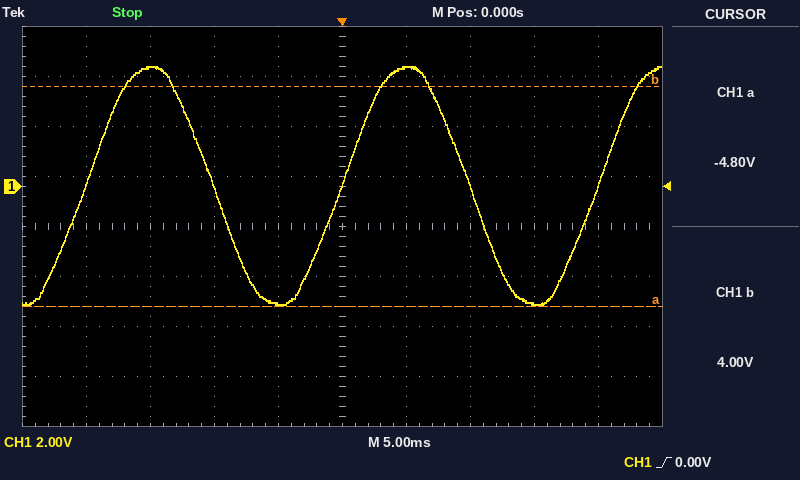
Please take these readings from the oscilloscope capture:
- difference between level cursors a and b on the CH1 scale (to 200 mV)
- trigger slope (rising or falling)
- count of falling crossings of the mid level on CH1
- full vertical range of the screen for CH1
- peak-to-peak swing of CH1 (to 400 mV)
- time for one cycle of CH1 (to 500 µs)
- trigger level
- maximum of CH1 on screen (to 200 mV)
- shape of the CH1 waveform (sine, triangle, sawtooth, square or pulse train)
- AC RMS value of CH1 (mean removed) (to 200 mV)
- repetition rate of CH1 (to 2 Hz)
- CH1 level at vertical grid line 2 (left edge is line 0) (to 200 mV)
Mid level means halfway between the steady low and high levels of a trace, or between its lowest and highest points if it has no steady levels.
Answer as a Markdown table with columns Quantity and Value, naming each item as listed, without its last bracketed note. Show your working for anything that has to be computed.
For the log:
| Quantity | Value |
|---|---|
| difference between level cursors a and b on the CH1 scale | 8.8 V |
| trigger slope | rising |
| count of falling crossings of the mid level on CH1 | 2 |
| full vertical range of the screen for CH1 | 16 V |
| peak-to-peak swing of CH1 | 9.6 V |
| time for one cycle of CH1 | 20.0 ms |
| trigger level | 0.00 V |
| maximum of CH1 on screen | 4.8 V |
| shape of the CH1 waveform | sine |
| AC RMS value of CH1 (mean removed) | 9.6 V / (2√2) ≈ 3.4 V |
| repetition rate of CH1 | 1 / 20.0 ms ≈ 50 Hz |
| CH1 level at vertical grid line 2 (left edge is line 0) | 4.8 V |
